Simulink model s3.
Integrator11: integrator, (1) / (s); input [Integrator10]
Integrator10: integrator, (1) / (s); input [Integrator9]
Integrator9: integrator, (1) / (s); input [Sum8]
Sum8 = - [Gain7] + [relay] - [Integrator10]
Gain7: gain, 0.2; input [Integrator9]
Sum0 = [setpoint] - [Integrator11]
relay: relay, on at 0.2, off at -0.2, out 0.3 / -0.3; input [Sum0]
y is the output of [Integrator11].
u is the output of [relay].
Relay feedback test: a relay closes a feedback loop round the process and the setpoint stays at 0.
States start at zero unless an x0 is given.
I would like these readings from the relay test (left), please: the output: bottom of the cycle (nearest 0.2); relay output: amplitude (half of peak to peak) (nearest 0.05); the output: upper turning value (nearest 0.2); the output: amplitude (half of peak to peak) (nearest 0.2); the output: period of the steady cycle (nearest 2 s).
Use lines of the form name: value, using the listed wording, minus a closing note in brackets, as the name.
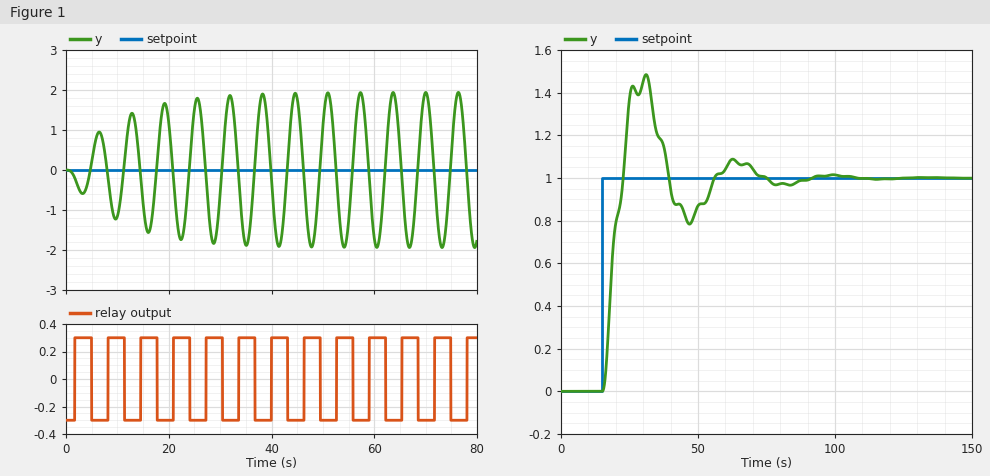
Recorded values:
the output: bottom of the cycle: -2.0
relay output: amplitude (half of peak to peak): 0.30
the output: upper turning value: 2.0
the output: amplitude (half of peak to peak): 2.0
the output: period of the steady cycle: 6 s
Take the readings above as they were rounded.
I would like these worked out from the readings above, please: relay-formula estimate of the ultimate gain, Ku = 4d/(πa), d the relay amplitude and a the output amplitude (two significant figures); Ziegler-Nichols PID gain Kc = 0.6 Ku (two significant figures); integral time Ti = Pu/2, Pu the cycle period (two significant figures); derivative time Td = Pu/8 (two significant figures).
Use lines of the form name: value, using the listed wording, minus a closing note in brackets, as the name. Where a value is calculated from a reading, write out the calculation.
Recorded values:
relay-formula estimate of the ultimate gain, Ku = 4d/(πa), d the relay amplitude and a the output amplitude: 4 × 0.3 / (π × 2) = 0.19
Ziegler-Nichols PID gain Kc = 0.6 Ku: 0.6 × 0.19 = 0.11
integral time Ti = Pu/2, Pu the cycle period: 6 / 2 = 3.0 s
derivative time Td = Pu/8: 6 / 8 = 0.75 s
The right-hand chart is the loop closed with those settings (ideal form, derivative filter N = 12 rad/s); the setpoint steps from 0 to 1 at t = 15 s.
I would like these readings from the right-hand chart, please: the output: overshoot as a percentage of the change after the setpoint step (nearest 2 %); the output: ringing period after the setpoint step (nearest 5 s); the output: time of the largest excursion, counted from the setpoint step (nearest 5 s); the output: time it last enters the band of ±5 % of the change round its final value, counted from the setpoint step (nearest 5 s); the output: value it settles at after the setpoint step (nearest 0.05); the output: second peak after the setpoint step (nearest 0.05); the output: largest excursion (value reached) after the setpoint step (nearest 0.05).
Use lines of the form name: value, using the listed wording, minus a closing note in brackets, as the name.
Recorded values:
the output: overshoot as a percentage of the change after the setpoint step: 48 %
the output: ringing period after the setpoint step: 30 s
the output: time of the largest excursion, counted from the setpoint step: 15 s
the output: time it last enters the band of ±5 % of the change round its final value, counted from the setpoint step: 55 s
the output: value it settles at after the setpoint step: 1.00
the output: second peak after the setpoint step: 1.10
the output: largest excursion (value reached) after the setpoint step: 1.50
